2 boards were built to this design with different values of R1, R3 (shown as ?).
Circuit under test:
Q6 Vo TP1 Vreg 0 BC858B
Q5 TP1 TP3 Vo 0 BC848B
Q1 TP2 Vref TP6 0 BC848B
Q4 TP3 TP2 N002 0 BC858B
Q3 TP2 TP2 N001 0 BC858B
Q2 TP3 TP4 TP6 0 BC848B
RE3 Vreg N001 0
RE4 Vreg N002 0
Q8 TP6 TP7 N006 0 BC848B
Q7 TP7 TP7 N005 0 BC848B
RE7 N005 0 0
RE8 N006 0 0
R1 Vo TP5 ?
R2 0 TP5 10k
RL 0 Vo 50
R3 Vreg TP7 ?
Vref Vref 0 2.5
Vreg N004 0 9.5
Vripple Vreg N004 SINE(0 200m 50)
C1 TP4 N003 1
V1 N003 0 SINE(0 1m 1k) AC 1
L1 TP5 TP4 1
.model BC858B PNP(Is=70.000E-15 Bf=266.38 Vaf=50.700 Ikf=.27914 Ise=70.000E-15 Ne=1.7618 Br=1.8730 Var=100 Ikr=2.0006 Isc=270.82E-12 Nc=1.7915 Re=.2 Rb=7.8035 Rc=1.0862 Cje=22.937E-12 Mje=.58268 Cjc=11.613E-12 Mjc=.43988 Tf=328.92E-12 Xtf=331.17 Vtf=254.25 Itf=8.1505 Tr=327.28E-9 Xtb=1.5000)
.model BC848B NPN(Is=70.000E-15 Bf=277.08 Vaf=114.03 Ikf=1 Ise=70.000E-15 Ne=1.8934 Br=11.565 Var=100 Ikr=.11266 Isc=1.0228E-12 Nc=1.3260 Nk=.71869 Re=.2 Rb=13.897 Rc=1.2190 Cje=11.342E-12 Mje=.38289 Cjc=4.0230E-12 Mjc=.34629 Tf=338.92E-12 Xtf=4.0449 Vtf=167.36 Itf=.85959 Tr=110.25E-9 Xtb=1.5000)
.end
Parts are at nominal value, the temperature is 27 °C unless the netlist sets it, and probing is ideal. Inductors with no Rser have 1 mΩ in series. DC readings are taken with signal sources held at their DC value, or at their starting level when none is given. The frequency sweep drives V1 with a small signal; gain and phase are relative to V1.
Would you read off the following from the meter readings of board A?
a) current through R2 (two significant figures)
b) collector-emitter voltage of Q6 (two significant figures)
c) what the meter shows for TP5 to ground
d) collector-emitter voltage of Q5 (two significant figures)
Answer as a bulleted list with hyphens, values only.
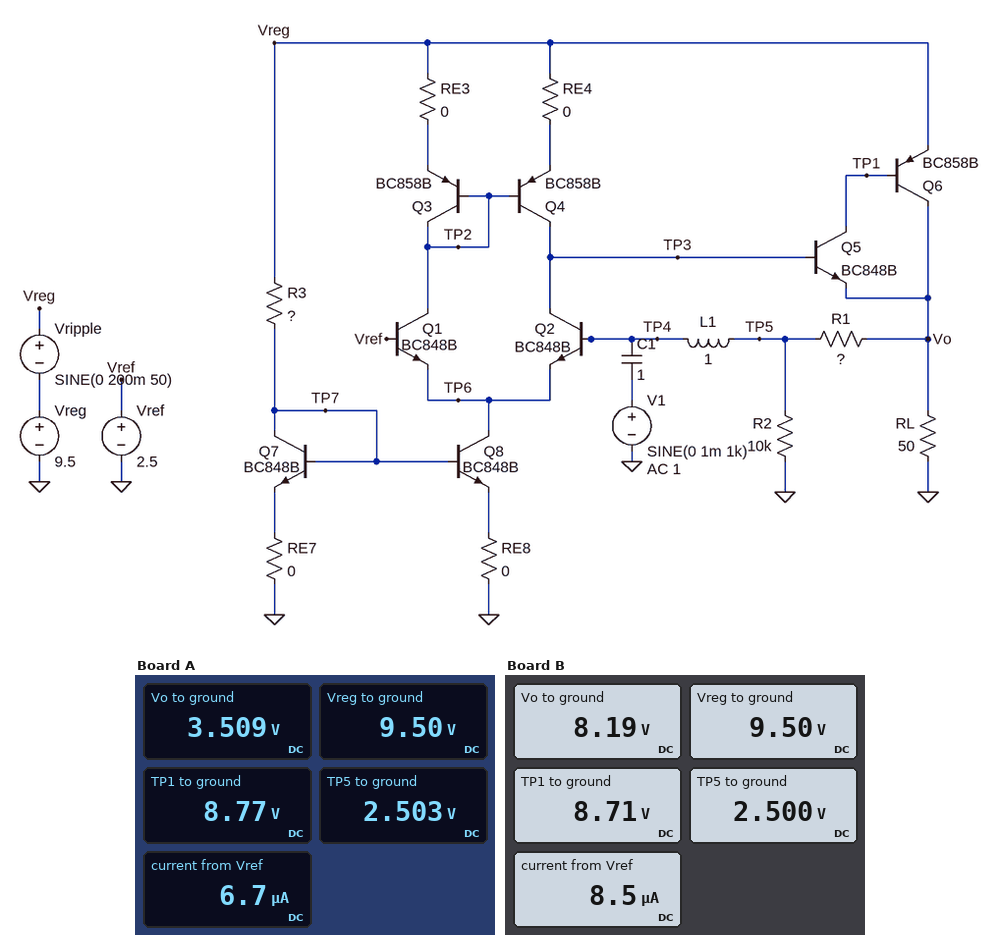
- 250 µA
- -6.0 V
- 2.503 V
- 5.3 V
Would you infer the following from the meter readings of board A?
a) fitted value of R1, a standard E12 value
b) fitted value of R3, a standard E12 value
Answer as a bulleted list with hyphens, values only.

- 3.9 kΩ
- 2.2 kΩ
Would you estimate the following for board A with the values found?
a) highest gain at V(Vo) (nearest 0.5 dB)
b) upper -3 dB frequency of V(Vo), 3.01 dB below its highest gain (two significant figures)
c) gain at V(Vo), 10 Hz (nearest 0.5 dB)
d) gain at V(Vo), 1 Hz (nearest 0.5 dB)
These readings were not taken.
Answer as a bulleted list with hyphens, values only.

- 63.0 dB
- 420 kHz
- 63.0 dB
- 63.0 dB
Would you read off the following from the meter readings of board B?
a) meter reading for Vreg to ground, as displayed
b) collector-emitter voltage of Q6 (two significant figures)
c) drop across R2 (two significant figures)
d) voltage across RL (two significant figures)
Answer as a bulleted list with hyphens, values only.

- 9.50 V
- -1.3 V
- 2.5 V
- 8.2 V
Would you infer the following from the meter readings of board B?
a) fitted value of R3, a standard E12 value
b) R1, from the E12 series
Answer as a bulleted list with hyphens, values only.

- 1.8 kΩ
- 22 kΩ
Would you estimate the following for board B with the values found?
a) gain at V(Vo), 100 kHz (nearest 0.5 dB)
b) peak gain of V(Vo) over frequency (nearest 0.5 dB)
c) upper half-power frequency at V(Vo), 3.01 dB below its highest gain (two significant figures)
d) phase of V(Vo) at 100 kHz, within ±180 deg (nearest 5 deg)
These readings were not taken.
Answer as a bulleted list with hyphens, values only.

- 62.0 dB
- 62.5 dB
- 280 kHz
- 160 deg
